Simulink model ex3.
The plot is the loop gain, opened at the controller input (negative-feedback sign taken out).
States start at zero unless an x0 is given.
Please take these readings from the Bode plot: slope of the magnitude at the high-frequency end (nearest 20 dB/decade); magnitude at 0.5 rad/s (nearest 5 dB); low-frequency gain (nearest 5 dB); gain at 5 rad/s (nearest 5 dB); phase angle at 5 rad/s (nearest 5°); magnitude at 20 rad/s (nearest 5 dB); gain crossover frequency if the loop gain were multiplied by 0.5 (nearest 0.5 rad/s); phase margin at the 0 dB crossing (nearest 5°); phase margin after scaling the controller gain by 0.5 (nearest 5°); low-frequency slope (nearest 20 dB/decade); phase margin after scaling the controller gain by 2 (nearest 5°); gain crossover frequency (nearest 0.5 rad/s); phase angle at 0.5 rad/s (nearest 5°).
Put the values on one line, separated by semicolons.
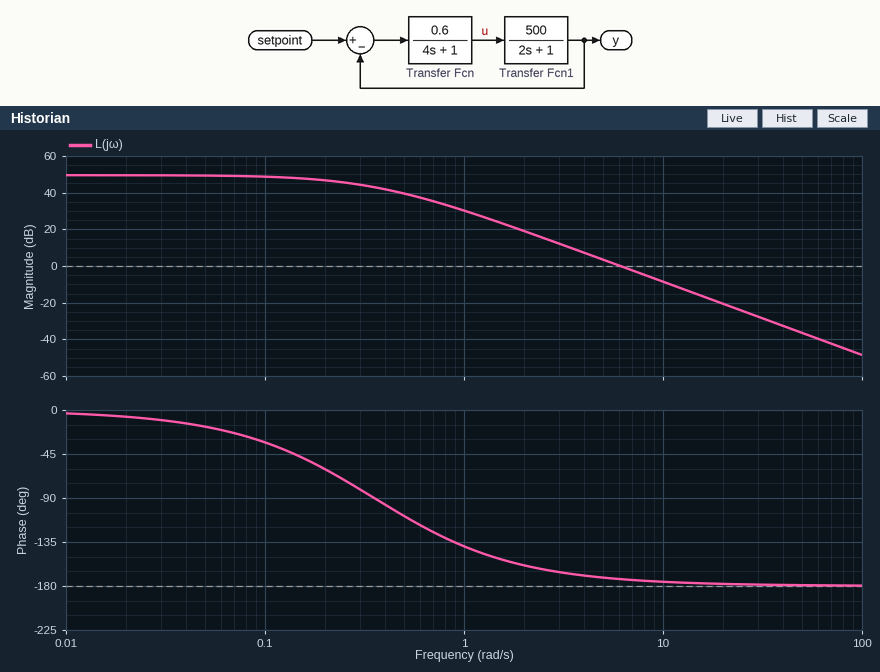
-40 dB/decade; 40 dB; 50 dB; 5 dB; -170°; -20 dB; 4.5 rad/s; 5°; 10°; 0 dB/decade; 5°; 6.0 rad/s; -110°
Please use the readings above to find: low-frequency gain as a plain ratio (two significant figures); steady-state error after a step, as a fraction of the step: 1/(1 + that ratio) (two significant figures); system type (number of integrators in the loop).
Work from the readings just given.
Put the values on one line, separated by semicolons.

320; 0.0031; 0
